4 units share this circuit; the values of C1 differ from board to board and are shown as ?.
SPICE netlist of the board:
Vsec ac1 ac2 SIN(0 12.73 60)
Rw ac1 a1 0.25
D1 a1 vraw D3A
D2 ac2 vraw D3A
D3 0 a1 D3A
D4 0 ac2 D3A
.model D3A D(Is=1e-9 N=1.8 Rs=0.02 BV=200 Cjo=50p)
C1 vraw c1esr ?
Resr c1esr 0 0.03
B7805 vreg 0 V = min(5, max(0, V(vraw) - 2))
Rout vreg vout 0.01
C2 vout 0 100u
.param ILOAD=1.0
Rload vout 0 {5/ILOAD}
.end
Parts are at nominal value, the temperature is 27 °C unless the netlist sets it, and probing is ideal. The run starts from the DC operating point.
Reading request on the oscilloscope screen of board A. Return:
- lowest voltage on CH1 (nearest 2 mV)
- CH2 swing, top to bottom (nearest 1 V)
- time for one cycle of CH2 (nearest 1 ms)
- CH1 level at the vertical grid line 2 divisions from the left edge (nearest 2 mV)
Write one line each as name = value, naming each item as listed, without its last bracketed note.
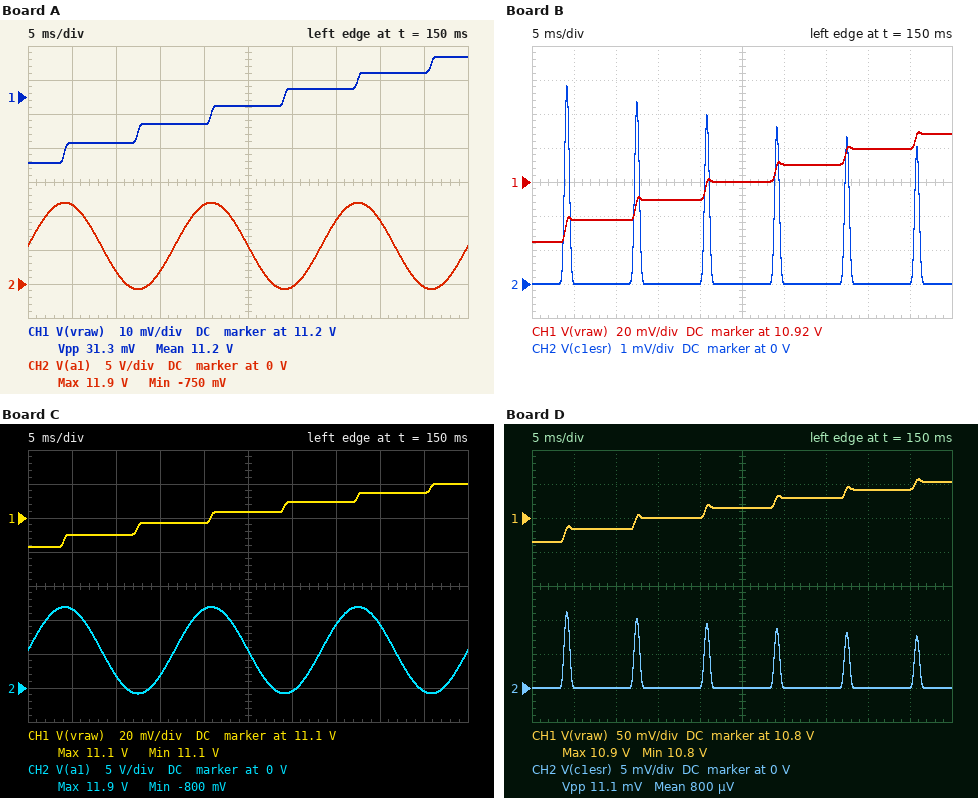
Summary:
lowest voltage on CH1 = 11.180 V
CH2 swing, top to bottom = 13 V
time for one cycle of CH2 = 17 ms
CH1 level at the vertical grid line 2 divisions from the left edge = 11.186 V
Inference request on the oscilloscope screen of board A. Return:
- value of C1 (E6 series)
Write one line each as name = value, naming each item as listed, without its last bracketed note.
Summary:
value of C1 = 1.5 mF
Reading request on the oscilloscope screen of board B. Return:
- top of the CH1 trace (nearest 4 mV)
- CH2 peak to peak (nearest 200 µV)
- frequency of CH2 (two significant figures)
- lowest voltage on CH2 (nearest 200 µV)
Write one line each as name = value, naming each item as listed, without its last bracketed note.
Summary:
top of the CH1 trace = 10.948 V
CH2 peak to peak = 5.8 mV
frequency of CH2 = 120 Hz
lowest voltage on CH2 = 0 V
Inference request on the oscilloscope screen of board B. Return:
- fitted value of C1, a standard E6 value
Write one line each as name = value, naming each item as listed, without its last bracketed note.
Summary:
fitted value of C1, a standard E6 value = 10 mF
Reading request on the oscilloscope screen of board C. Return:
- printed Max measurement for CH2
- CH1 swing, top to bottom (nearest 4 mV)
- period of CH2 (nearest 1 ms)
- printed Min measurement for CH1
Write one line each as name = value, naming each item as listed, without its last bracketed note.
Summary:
printed Max measurement for CH2 = 11.9 V
CH1 swing, top to bottom = 36 mV
period of CH2 = 17 ms
printed Min measurement for CH1 = 11.1 V
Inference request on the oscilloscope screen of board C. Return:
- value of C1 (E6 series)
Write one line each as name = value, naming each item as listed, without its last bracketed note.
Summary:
value of C1 = 3.3 mF
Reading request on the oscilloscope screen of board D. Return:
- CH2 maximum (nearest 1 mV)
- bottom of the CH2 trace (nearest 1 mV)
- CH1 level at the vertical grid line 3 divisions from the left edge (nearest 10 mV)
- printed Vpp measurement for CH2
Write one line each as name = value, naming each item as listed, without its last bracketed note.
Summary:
CH2 maximum = 11 mV
bottom of the CH2 trace = 0 V
CH1 level at the vertical grid line 3 divisions from the left edge = 10.80 V
printed Vpp measurement for CH2 = 11.1 mV
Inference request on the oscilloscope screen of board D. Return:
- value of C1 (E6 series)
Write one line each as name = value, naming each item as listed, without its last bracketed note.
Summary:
value of C1 = 15 mF
